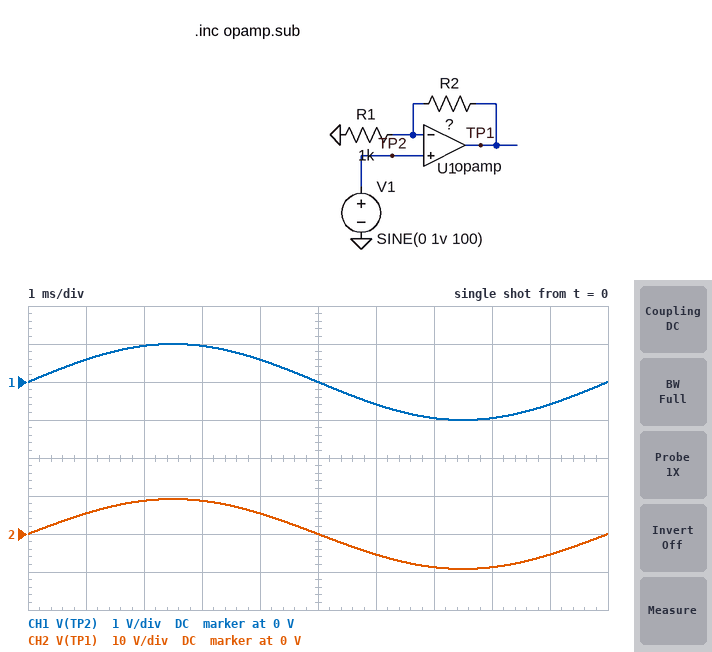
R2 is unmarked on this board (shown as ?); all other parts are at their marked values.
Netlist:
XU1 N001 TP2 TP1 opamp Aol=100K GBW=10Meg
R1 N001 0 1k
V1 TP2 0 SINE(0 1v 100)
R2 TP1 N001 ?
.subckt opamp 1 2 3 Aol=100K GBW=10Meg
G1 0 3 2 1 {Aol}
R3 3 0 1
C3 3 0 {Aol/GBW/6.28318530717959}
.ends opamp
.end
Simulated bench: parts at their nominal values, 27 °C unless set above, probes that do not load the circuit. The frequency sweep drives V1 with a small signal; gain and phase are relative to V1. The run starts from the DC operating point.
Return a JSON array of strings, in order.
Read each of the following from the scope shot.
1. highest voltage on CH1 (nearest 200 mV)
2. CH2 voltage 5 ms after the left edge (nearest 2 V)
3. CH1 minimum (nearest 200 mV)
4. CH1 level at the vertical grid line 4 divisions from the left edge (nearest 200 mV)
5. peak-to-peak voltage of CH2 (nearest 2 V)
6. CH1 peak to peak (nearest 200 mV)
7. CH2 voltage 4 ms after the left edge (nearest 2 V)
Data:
["1.0 V", "0 V", "-1.0 V", "600 mV", "18 V", "2.0 V", "6 V"]
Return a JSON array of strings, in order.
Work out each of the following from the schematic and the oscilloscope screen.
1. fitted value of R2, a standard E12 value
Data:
["8.2 kΩ"]
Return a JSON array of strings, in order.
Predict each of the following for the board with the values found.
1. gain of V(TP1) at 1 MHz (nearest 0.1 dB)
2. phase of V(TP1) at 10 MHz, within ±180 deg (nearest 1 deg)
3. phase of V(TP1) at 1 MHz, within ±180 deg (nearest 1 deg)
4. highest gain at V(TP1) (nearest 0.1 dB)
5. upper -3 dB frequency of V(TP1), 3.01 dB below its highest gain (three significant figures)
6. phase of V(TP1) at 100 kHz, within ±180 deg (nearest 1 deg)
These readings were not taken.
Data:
["16.6 dB", "-84 deg", "-43 deg", "19.3 dB", "1.09 MHz", "-5 deg"]
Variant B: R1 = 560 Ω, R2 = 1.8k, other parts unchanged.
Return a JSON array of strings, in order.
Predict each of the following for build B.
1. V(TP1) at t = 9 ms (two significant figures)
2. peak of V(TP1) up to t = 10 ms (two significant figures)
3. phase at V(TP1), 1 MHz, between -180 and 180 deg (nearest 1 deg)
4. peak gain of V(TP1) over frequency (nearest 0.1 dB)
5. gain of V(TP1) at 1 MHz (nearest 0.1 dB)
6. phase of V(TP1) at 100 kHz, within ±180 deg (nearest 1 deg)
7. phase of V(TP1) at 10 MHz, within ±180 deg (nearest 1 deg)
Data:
["-2.5 V", "4.2 V", "-23 deg", "12.5 dB", "11.8 dB", "-2 deg", "-77 deg"]
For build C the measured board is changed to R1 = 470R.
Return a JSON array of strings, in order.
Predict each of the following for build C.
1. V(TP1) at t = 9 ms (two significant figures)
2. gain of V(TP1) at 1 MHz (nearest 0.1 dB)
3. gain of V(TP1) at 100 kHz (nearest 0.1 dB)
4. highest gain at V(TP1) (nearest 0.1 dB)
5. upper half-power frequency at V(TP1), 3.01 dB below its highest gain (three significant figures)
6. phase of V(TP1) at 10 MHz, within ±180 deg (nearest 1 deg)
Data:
["-11 V", "18.9 dB", "25.2 dB", "25.3 dB", "542 kHz", "-87 deg"]
